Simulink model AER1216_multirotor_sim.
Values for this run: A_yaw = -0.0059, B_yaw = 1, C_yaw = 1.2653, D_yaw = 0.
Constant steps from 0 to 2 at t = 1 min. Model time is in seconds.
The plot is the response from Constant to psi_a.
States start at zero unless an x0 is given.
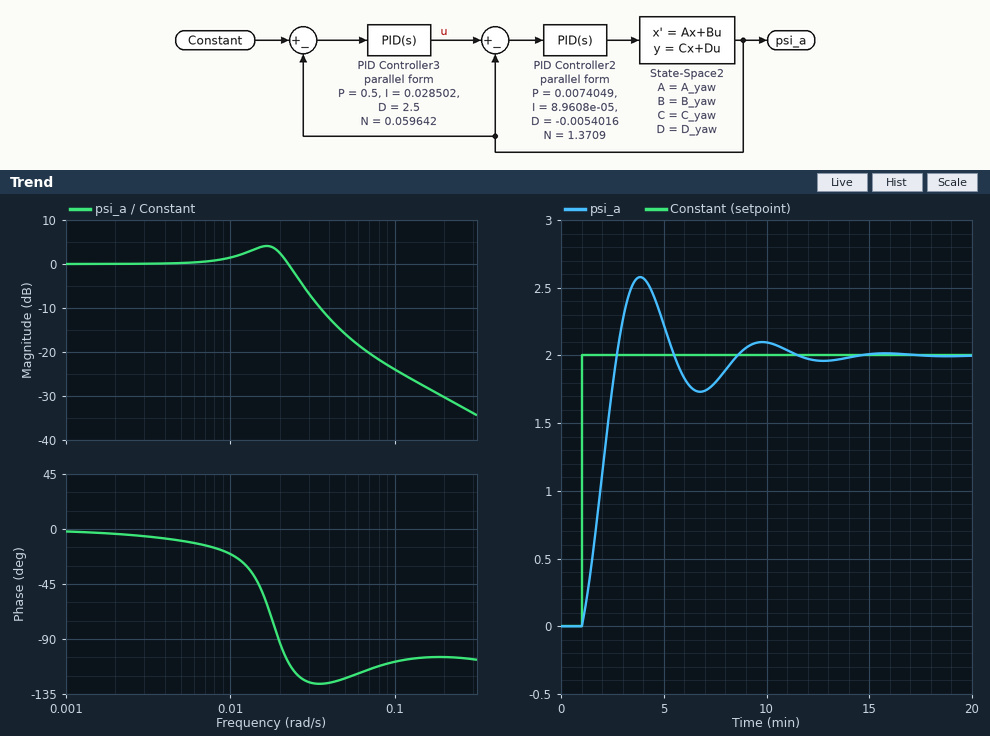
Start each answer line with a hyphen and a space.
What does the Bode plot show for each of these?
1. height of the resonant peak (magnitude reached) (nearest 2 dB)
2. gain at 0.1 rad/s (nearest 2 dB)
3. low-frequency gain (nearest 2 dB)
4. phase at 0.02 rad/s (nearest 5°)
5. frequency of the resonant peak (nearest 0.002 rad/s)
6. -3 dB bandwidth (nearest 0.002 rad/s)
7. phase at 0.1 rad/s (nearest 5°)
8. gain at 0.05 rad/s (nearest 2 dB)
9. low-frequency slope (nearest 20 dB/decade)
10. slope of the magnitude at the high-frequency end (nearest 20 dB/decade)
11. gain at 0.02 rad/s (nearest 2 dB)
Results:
- 4 dB
- -24 dB
- 0 dB
- -95°
- 0.016 rad/s
- 0.026 rad/s
- -110°
- -16 dB
- 0 dB/decade
- -20 dB/decade
- 2 dB
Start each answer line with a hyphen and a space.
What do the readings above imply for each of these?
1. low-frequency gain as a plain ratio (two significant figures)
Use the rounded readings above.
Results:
- 1.0
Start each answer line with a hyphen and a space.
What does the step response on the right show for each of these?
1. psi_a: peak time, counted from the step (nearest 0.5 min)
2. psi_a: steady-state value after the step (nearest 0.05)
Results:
- 3.0 min
- 2.00
